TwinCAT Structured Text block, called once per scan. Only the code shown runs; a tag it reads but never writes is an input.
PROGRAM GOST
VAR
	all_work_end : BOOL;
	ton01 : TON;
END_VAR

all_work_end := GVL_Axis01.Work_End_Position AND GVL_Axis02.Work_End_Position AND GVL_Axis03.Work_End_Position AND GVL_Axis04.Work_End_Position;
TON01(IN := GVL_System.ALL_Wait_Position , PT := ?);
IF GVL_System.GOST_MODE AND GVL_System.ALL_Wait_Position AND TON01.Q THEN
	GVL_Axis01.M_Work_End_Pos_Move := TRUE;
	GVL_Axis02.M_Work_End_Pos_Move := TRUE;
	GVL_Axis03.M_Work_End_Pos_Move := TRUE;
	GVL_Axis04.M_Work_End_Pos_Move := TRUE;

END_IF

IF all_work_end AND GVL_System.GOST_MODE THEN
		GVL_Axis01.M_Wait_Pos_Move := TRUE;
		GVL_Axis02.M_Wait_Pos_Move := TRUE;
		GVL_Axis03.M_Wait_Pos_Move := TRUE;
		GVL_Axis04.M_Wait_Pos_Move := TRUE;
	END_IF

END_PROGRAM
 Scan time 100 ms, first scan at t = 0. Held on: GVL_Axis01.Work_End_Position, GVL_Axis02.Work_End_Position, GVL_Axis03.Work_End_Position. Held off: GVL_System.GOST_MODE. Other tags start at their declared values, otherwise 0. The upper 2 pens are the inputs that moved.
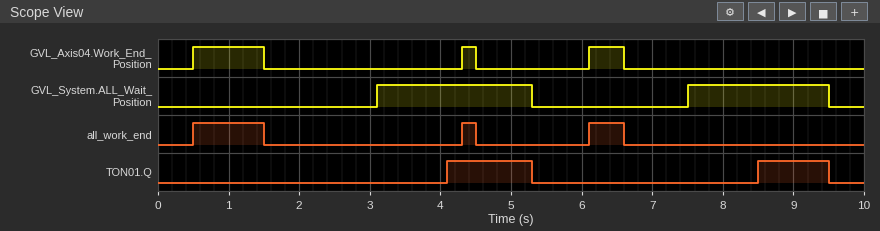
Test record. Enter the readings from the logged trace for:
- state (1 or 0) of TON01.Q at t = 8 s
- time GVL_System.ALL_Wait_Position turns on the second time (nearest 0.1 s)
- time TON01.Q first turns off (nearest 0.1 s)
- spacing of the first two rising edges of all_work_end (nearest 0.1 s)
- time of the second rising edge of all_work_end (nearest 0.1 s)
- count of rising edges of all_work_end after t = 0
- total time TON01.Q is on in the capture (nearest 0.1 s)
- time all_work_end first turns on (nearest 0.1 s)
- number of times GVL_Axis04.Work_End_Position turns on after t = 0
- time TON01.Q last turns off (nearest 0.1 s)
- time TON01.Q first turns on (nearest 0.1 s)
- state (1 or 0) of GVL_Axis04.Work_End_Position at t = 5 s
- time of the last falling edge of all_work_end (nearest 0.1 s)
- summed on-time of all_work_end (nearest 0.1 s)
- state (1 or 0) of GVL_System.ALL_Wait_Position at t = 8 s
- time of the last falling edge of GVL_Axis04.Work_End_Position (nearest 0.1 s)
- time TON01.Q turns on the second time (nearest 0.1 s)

0
7.5 s
5.3 s
3.8 s
4.3 s
3
2.2 s
0.5 s
3
9.5 s
4.1 s
0
6.6 s
1.7 s
1
6.6 s
8.5 s
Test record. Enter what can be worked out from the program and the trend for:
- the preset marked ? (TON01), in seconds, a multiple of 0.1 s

1.0 s
